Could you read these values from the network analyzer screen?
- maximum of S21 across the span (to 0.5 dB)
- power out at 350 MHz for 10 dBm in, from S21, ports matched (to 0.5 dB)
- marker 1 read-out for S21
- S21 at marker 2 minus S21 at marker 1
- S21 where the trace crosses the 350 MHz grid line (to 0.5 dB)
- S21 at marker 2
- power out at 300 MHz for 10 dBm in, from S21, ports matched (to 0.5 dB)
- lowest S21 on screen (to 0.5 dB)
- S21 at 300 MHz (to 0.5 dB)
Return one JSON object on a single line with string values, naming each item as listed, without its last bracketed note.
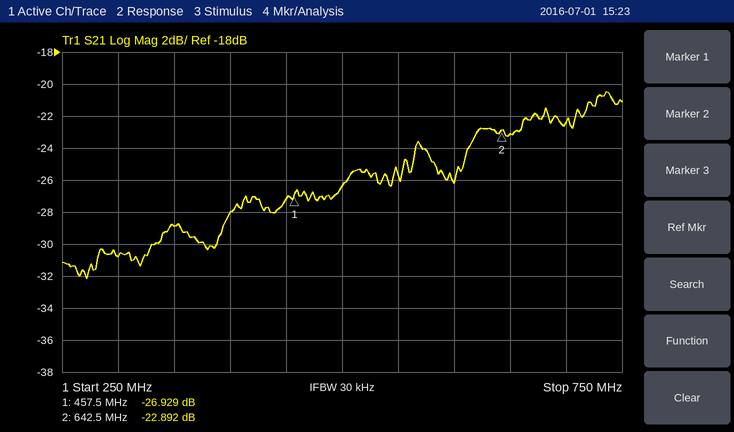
{"maximum of S21 across the span": "-20.5 dB", "power out at 350 MHz for 10 dBm in, from S21, ports matched": "-19.0 dBm", "marker 1 read-out for S21": "-26.929 dB", "S21 at marker 2 minus S21 at marker 1": "4.037 dB", "S21 where the trace crosses the 350 MHz grid line": "-29.0 dB", "S21 at marker 2": "-22.892 dB", "power out at 300 MHz for 10 dBm in, from S21, ports matched": "-21.0 dBm", "lowest S21 on screen": "-32.0 dB", "S21 at 300 MHz": "-31.0 dB"}
